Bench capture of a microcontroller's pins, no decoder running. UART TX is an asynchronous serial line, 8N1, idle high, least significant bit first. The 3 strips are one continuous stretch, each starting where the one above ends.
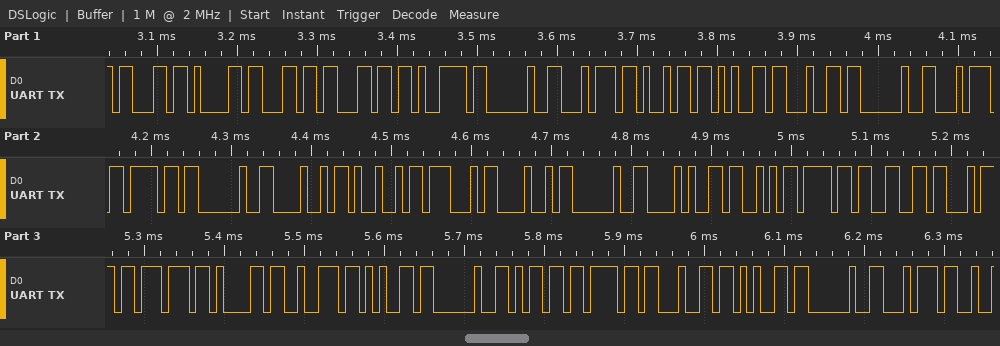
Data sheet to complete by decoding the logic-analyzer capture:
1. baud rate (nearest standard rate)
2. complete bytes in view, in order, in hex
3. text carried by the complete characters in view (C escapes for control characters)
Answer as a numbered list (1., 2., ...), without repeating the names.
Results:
1. 115200 baud
2. 63 61 6C 6C 79 20 74 69 65 64 20 74 6F 20 48 49 47 48 20 28 53 6F 66 74 77 61 72 65 20 6D 6F 64 65 20 74
3. "cally tied to HIGH (Software mode t"
